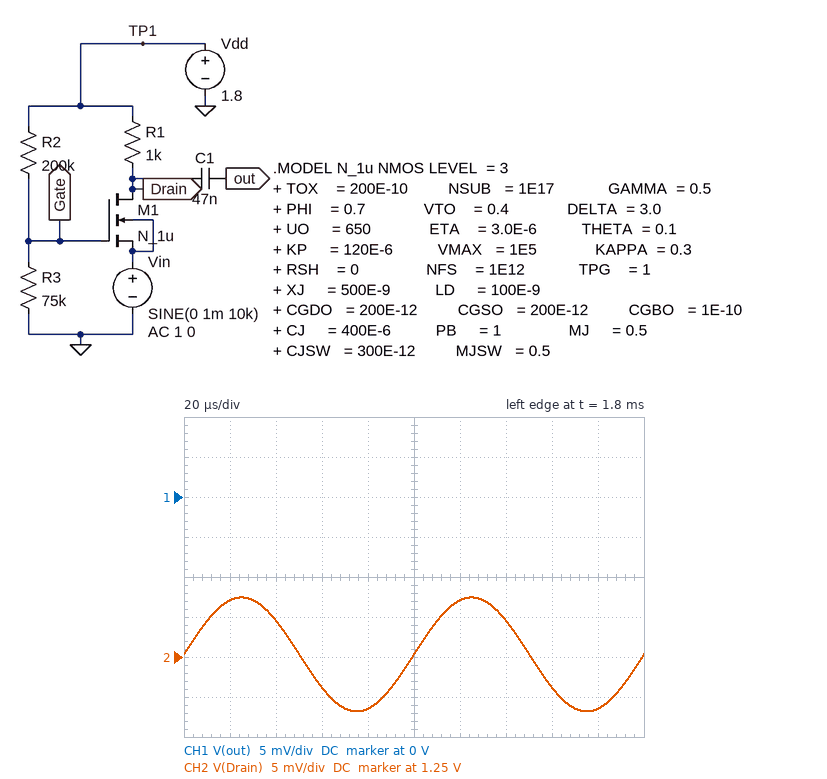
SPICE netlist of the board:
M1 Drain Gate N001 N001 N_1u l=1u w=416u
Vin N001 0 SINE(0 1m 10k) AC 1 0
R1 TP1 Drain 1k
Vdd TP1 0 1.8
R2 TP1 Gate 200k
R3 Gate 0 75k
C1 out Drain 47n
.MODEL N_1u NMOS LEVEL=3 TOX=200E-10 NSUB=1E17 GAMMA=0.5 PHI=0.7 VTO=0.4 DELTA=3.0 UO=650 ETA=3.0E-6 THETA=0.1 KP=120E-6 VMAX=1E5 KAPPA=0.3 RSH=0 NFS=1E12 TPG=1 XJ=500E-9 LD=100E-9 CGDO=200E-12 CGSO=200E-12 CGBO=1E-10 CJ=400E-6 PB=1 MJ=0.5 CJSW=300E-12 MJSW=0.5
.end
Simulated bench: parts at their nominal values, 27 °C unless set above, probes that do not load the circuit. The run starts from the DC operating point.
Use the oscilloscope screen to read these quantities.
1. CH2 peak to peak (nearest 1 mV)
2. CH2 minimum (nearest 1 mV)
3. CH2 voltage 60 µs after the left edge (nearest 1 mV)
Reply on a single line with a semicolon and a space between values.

14 mV; 1.243 V; 1.246 V
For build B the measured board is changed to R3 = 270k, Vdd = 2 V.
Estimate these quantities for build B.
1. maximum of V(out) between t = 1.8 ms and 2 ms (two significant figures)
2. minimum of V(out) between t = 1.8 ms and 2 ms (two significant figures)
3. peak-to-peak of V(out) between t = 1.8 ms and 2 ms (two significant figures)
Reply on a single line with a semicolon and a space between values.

46 mV; 44 mV; 2.1 mV
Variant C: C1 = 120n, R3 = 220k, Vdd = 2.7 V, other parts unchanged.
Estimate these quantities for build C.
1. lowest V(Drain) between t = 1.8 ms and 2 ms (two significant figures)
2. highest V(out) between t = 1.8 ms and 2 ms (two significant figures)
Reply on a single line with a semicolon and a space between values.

46 mV; 48 mV
